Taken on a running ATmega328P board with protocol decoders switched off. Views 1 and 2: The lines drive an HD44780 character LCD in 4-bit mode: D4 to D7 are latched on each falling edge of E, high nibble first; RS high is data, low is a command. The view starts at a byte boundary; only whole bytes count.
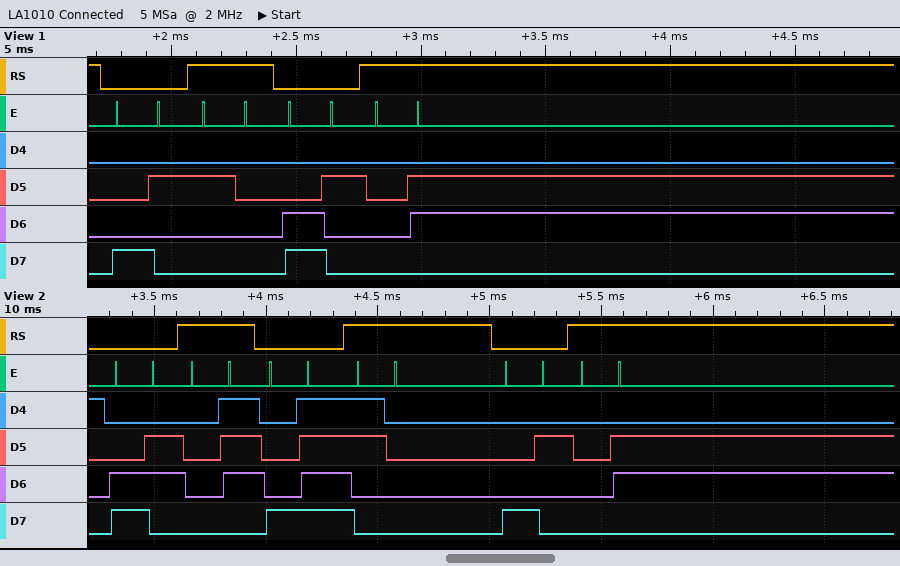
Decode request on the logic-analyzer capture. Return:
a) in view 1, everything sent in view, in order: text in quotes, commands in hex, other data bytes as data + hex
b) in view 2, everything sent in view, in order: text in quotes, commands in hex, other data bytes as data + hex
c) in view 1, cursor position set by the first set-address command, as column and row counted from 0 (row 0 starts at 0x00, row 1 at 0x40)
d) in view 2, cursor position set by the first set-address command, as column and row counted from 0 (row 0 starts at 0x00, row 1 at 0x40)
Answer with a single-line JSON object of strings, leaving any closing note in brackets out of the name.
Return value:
{"in view 1, everything sent in view, in order: text in quotes, commands in hex, other data bytes as data + hex": "0x82 \" \" 0xC2 data 06", "in view 2, everything sent in view, in order: text in quotes, commands in hex, other data bytes as data + hex": "0xC6 data 07 0x8F \"0\" 0x82 data 06", "in view 1, cursor position set by the first set-address command, as column and row counted from 0": "column 2, row 0", "in view 2, cursor position set by the first set-address command, as column and row counted from 0": "column 6, row 1"}
